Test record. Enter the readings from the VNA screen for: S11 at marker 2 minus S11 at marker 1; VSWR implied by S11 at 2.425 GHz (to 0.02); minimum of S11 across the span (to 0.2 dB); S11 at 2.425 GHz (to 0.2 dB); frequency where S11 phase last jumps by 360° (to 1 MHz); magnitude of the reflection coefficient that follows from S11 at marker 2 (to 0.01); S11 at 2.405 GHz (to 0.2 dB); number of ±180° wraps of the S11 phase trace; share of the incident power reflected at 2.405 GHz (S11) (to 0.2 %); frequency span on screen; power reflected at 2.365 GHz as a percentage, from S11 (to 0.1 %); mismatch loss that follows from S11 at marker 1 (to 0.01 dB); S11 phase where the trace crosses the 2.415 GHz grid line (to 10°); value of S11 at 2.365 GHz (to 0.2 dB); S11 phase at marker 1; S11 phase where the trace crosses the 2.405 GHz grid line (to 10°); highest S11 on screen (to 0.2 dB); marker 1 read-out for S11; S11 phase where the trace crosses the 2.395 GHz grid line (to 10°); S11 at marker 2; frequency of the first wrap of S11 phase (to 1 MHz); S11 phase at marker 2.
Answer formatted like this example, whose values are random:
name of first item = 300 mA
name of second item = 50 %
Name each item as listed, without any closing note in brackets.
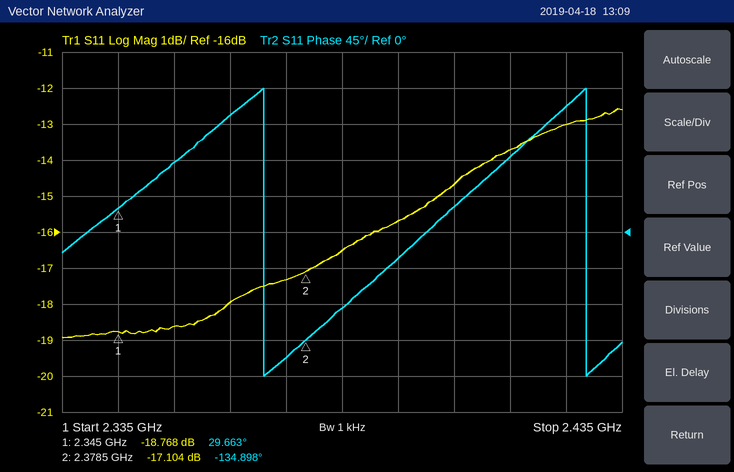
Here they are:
S11 at marker 2 minus S11 at marker 1 = 1.664 dB
VSWR implied by S11 at 2.425 GHz = 1.58
minimum of S11 across the span = -19.0 dB
S11 at 2.425 GHz = -13.0 dB
frequency where S11 phase last jumps by 360° = 2.429 GHz
magnitude of the reflection coefficient that follows from S11 at marker 2 = 0.14
S11 at 2.405 GHz = -14.6 dB
number of ±180° wraps of the S11 phase trace = 2
share of the incident power reflected at 2.405 GHz (S11) = 3.4 %
frequency span on screen = 100 MHz
power reflected at 2.365 GHz as a percentage, from S11 = 1.6 %
mismatch loss that follows from S11 at marker 1 = 0.06 dB
S11 phase where the trace crosses the 2.415 GHz grid line = 90°
value of S11 at 2.365 GHz = -18.0 dB
S11 phase at marker 1 = 29.663°
S11 phase where the trace crosses the 2.405 GHz grid line = 30°
highest S11 on screen = -12.6 dB
marker 1 read-out for S11 = -18.768 dB
S11 phase where the trace crosses the 2.395 GHz grid line = -30°
S11 at marker 2 = -17.104 dB
frequency of the first wrap of S11 phase = 2.371 GHz
S11 phase at marker 2 = -134.898°
